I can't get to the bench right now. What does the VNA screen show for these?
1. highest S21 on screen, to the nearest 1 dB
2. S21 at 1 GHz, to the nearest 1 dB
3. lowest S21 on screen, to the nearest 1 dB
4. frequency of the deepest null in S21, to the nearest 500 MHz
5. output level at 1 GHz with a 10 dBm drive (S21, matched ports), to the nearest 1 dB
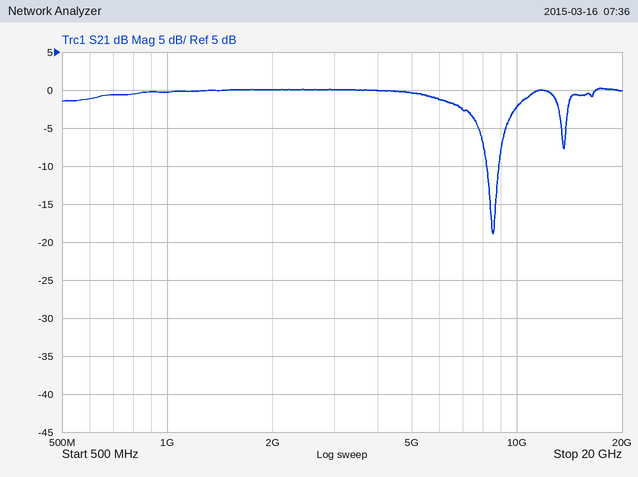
0 dB
0 dB
-19 dB
8.5 GHz
10 dBm
